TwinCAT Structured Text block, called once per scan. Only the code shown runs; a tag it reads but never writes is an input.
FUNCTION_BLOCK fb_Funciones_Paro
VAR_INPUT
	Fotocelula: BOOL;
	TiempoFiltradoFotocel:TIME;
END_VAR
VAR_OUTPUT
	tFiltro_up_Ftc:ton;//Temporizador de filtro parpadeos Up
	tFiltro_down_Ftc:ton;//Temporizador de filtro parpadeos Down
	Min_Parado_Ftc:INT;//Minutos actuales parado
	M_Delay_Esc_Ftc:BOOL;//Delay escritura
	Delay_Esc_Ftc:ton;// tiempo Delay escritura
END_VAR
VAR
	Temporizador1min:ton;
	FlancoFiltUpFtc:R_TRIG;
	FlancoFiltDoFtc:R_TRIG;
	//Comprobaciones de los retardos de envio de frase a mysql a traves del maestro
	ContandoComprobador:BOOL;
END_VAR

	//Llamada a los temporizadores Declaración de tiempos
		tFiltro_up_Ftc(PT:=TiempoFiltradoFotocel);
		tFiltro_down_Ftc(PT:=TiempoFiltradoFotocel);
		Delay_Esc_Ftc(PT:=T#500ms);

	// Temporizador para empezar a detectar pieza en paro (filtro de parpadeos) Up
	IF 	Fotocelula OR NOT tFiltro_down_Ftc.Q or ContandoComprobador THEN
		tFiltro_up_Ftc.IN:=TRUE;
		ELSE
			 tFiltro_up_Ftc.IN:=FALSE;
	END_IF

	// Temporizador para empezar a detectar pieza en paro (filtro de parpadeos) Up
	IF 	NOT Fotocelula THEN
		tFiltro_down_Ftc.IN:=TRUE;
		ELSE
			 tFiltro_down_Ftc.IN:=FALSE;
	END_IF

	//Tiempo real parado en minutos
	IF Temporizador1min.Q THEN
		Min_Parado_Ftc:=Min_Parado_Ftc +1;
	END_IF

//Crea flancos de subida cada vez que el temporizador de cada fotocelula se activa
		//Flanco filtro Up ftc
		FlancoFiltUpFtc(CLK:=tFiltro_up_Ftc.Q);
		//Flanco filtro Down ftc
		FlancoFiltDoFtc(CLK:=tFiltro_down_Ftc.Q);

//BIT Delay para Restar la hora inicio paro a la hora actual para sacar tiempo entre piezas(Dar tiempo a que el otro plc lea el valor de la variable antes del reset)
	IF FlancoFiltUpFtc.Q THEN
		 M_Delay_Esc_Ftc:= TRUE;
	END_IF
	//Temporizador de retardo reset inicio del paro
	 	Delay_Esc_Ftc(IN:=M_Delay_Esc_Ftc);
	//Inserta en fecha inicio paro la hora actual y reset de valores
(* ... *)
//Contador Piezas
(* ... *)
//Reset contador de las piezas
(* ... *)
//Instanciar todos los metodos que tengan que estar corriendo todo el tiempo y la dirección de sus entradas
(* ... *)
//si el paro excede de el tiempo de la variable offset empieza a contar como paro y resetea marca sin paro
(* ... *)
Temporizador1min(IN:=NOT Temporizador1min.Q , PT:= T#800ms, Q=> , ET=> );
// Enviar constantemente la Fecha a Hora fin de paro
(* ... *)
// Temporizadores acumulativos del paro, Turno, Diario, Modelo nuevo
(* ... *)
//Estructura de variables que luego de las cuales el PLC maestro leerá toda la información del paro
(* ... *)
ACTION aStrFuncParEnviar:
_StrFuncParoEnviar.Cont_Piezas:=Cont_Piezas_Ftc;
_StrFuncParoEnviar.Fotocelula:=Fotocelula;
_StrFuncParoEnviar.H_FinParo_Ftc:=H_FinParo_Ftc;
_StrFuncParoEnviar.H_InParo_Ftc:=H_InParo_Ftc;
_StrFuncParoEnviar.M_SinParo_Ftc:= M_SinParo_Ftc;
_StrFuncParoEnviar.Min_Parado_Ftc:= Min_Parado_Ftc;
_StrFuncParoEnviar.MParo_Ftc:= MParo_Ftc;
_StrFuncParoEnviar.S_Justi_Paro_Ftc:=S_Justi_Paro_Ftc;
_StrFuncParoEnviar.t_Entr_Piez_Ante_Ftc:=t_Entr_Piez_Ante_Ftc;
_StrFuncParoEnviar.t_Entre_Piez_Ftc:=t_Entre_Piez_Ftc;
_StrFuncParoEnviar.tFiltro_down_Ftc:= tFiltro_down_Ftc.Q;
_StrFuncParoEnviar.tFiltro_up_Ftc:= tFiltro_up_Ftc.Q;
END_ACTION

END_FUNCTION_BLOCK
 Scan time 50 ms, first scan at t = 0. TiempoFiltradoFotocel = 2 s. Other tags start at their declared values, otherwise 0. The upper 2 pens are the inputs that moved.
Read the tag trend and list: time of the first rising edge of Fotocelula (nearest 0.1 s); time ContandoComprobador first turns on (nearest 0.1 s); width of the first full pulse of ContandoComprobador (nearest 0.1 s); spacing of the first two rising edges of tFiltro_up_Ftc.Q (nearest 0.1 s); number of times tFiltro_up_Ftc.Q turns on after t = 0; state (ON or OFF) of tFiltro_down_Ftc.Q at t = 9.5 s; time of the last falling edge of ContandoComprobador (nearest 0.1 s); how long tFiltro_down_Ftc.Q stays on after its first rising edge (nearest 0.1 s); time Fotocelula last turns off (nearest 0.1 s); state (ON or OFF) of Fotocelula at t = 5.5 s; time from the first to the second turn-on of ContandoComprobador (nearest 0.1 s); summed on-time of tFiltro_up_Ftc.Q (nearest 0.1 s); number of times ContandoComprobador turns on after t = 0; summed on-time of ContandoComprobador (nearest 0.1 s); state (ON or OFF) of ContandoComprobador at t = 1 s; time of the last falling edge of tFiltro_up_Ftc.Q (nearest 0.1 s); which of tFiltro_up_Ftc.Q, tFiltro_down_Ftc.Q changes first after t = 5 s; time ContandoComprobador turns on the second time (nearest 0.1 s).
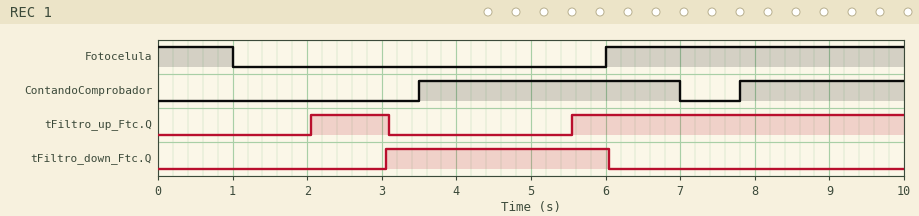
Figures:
6.0 s
3.5 s
3.5 s
3.5 s
2
OFF
7.0 s
3.0 s
1.0 s
OFF
4.3 s
5.5 s
2
5.7 s
OFF
3.1 s
tFiltro_up_Ftc.Q
7.8 s
